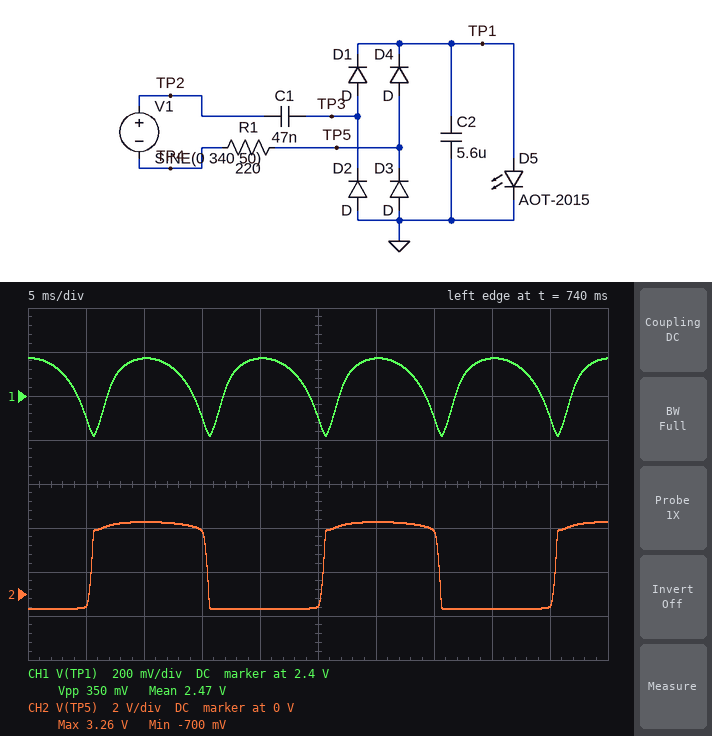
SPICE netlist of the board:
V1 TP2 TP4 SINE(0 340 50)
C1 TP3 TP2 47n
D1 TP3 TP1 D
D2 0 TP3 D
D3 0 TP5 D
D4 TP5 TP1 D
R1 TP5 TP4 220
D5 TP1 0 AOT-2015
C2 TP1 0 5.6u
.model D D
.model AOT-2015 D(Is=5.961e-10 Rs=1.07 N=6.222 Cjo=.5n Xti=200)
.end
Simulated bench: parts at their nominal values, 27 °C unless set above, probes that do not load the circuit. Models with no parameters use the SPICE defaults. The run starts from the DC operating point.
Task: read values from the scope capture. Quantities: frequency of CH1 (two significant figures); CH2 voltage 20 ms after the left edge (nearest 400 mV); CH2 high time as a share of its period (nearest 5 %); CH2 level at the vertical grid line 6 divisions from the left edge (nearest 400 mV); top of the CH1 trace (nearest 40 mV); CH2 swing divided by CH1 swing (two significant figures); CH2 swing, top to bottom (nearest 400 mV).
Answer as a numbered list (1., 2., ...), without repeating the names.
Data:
1. 100 Hz
2. -800 mV
3. 50 %
4. 3.2 V
5. 2.56 V
6. 11
7. 4.0 V
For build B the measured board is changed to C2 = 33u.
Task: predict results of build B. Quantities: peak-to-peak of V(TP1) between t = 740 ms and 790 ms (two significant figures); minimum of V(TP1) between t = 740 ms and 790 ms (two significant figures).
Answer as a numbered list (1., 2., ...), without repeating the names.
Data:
1. 160 mV
2. 2.4 V
